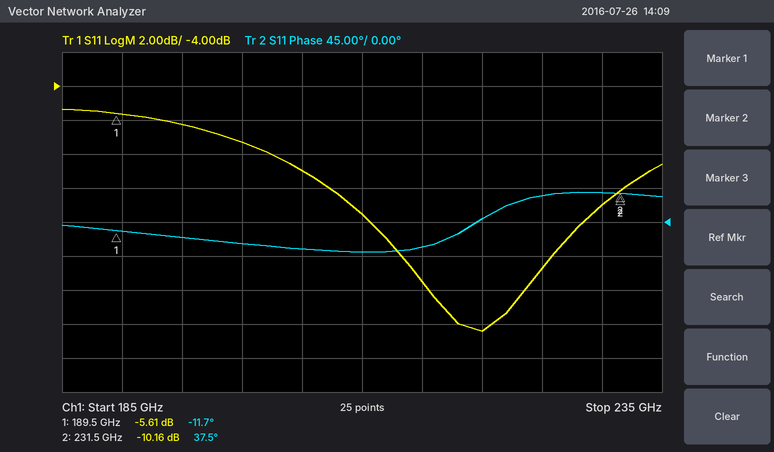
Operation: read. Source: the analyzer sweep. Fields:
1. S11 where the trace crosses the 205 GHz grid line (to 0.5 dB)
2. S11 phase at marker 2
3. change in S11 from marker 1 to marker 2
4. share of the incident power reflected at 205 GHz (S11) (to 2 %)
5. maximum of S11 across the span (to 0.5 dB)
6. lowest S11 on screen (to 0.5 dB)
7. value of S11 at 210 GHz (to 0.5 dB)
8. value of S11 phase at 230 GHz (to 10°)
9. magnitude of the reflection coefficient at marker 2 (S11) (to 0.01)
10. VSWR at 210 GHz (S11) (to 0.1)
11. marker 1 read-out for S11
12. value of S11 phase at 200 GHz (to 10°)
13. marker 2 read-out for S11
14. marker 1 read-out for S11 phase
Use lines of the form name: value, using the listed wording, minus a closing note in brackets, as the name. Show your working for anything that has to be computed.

S11 where the trace crosses the 205 GHz grid line: -9.0 dB
S11 phase at marker 2: 37.5°
change in S11 from marker 1 to marker 2: -10.16 − (-5.61) = -4.55 dB
share of the incident power reflected at 205 GHz (S11): 10^(-9/10) ≈ 12.6 %, so 12 % to the nearest 2 %
maximum of S11 across the span: -5.5 dB
lowest S11 on screen: -18.5 dB
value of S11 at 210 GHz: -11.5 dB
value of S11 phase at 230 GHz: 40°
magnitude of the reflection coefficient at marker 2 (S11): 10^(-10.16/20) ≈ 0.31
VSWR at 210 GHz (S11): |Γ| = 10^(-11.5/20) = 0.2661; VSWR = (1 + 0.2661)/(1 − 0.2661) ≈ 1.7
marker 1 read-out for S11: -5.61 dB
value of S11 phase at 200 GHz: -30°
marker 2 read-out for S11: -10.16 dB
marker 1 read-out for S11 phase: -11.7°
